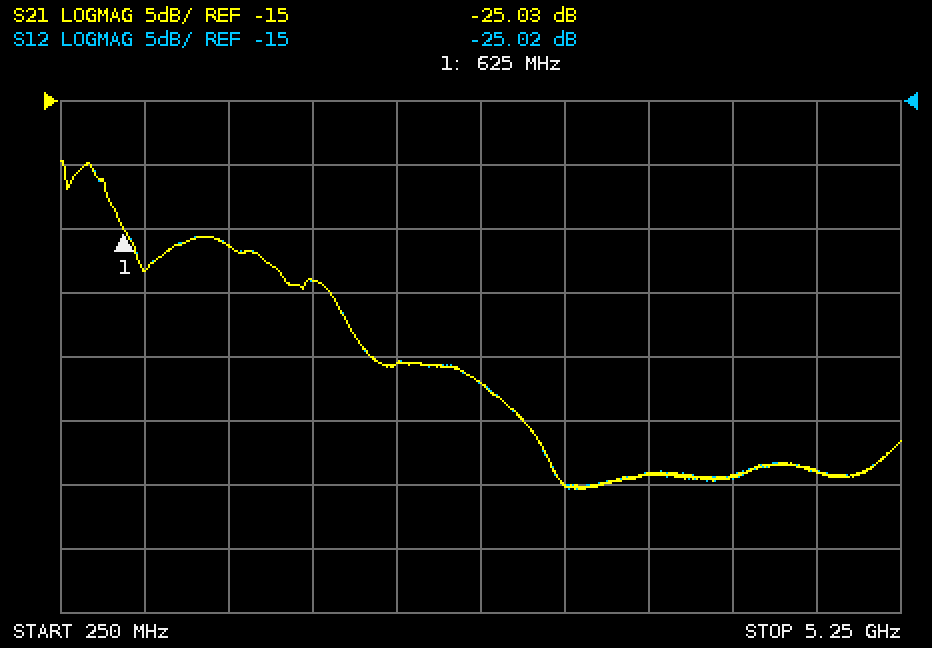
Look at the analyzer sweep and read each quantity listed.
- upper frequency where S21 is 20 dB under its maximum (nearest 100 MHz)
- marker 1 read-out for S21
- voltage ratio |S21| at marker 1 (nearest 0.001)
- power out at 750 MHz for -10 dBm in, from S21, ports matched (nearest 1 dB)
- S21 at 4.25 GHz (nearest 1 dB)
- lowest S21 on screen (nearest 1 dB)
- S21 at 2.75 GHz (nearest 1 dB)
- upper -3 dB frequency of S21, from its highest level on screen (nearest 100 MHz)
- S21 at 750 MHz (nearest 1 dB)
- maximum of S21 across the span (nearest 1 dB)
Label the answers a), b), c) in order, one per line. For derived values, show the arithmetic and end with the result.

a) 3.0 GHz
b) -25.03 dB
c) 10^(-25.03/20) ≈ 0.056
d) -10 dBm + (-28 dB) = -38 dBm
e) -44 dB
f) -45 dB
g) -37 dB
h) 500 MHz
i) -28 dB
j) -20 dB
